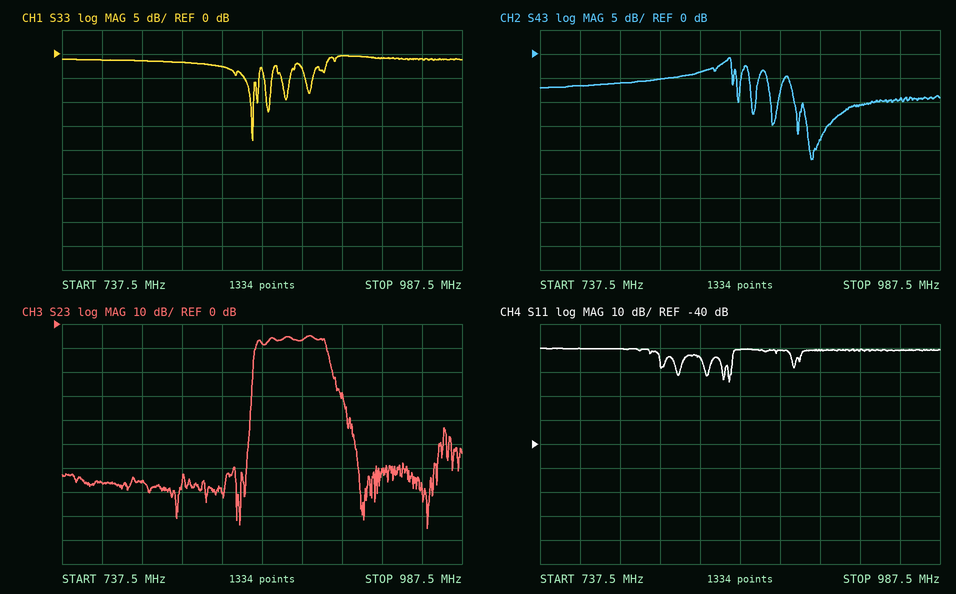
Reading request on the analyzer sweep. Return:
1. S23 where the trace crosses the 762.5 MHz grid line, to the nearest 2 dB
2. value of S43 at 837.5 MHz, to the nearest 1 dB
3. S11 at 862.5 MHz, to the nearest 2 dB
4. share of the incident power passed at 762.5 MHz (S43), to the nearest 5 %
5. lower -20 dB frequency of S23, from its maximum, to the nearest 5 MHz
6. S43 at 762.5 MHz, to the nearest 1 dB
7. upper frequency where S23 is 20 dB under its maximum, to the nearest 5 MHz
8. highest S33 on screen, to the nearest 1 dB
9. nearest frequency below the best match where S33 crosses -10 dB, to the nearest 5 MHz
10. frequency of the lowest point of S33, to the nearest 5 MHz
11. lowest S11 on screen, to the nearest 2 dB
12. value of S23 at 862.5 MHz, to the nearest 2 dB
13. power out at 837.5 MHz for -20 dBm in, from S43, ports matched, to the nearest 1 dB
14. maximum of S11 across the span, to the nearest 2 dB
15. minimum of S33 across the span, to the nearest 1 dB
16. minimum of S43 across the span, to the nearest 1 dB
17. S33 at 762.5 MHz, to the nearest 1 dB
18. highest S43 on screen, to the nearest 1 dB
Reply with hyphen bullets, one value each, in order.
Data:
- -66 dB
- -4 dB
- 0 dB
- 20 %
- 855 MHz
- -7 dB
- 910 MHz
- 0 dB
- 855 MHz
- 855 MHz
- -14 dB
- -8 dB
- -24 dBm
- 0 dB
- -18 dB
- -22 dB
- -1 dB
- -1 dB
